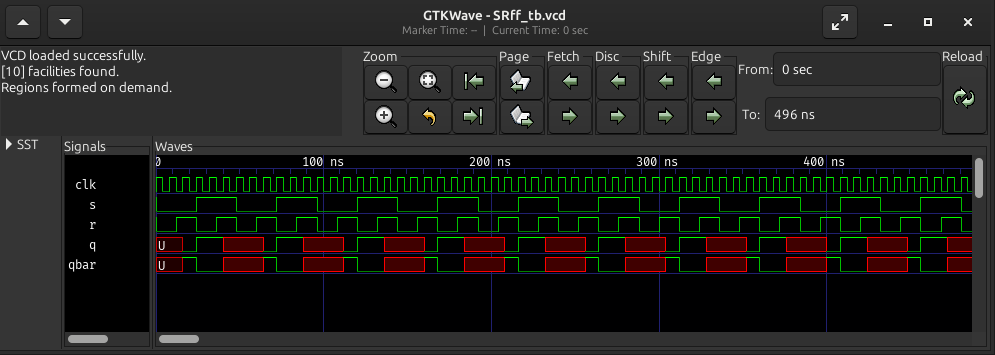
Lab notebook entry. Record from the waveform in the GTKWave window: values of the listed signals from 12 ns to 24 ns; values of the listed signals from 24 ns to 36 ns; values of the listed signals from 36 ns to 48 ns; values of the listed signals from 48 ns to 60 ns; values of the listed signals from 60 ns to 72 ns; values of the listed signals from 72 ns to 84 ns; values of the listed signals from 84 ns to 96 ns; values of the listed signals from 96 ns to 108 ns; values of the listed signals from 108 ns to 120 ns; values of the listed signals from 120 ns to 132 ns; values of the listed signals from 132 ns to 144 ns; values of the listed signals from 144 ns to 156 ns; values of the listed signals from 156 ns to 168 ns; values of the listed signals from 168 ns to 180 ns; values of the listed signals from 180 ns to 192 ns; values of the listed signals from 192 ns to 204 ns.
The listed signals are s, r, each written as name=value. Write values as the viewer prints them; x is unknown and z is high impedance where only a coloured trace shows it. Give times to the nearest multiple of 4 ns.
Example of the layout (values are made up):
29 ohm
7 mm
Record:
s=0, r=1
s=1, r=0
s=1, r=1
s=0, r=0
s=0, r=1
s=1, r=0
s=1, r=1
s=0, r=0
s=0, r=1
s=1, r=0
s=1, r=1
s=0, r=0
s=0, r=1
s=1, r=0
s=1, r=1
s=0, r=0
